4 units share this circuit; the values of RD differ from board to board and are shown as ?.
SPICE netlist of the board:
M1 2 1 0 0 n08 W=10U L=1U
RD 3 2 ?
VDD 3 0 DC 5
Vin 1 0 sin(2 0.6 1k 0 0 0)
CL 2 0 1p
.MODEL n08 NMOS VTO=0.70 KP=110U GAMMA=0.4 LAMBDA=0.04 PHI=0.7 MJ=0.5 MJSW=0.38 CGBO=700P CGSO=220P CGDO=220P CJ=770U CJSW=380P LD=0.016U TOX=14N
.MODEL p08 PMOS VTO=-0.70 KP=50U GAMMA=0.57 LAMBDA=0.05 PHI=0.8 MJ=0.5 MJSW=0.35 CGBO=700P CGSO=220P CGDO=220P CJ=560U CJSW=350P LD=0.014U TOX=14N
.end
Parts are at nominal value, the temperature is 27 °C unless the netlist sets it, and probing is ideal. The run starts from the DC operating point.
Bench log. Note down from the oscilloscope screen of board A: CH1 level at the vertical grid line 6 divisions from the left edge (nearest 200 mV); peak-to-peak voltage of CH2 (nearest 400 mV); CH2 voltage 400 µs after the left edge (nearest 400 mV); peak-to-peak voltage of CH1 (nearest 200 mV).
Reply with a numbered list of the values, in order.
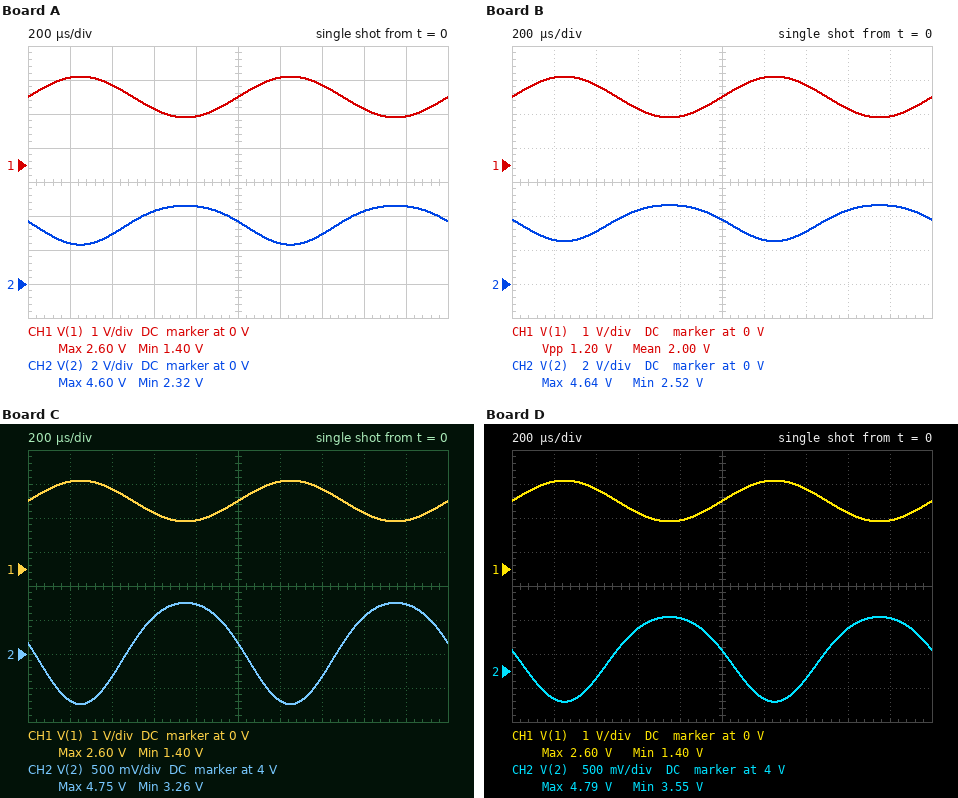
1. 2.6 V
2. 2.4 V
3. 2.8 V
4. 1.2 V
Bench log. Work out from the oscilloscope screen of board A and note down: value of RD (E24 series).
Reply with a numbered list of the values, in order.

1. 1.2 kΩ
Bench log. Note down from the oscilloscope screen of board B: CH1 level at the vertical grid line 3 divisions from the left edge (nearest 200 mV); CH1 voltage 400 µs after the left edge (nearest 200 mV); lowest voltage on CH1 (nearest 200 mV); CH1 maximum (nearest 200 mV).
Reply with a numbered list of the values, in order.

1. 1.6 V
2. 2.4 V
3. 1.4 V
4. 2.6 V
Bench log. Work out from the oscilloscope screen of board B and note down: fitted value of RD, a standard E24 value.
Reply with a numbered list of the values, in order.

1. 1.1 kΩ
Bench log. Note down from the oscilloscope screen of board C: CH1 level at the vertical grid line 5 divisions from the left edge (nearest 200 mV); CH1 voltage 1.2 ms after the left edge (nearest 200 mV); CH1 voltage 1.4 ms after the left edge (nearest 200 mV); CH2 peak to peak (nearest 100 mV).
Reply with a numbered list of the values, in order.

1. 2.0 V
2. 2.6 V
3. 2.4 V
4. 1.5 V
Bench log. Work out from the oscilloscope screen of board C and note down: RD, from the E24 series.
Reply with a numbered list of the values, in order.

1. 750 Ω
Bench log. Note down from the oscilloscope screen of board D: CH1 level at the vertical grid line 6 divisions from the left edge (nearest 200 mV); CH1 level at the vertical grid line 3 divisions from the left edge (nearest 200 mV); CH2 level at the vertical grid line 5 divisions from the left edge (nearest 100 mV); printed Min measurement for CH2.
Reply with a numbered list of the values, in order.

1. 2.6 V
2. 1.6 V
3. 4.3 V
4. 3.55 V
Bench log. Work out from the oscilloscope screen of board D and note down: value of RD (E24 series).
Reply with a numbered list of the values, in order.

1. 620 Ω
